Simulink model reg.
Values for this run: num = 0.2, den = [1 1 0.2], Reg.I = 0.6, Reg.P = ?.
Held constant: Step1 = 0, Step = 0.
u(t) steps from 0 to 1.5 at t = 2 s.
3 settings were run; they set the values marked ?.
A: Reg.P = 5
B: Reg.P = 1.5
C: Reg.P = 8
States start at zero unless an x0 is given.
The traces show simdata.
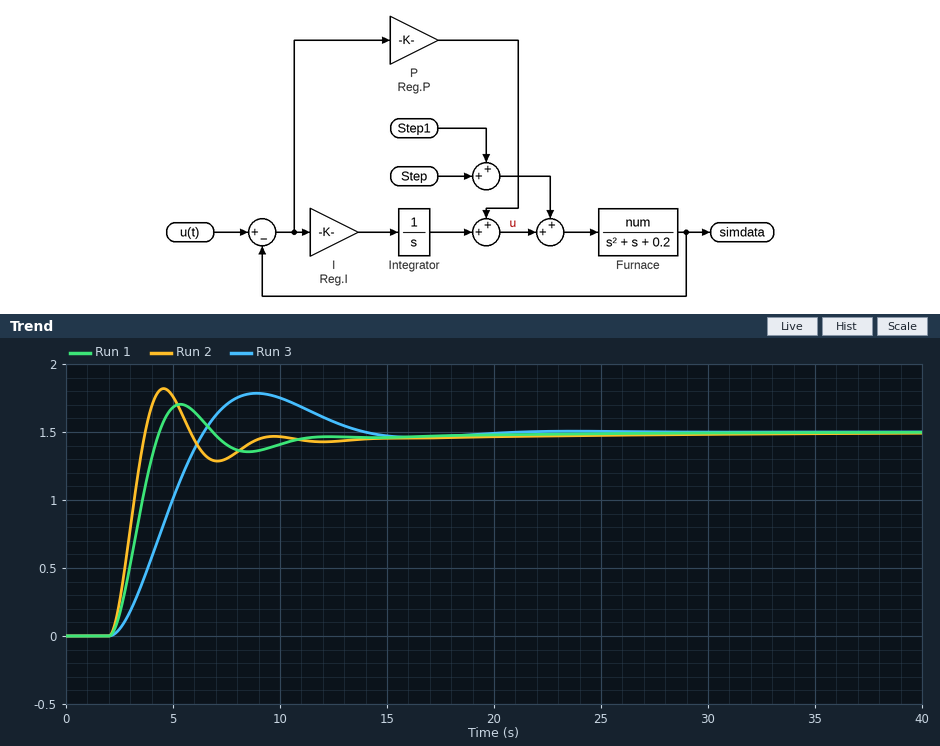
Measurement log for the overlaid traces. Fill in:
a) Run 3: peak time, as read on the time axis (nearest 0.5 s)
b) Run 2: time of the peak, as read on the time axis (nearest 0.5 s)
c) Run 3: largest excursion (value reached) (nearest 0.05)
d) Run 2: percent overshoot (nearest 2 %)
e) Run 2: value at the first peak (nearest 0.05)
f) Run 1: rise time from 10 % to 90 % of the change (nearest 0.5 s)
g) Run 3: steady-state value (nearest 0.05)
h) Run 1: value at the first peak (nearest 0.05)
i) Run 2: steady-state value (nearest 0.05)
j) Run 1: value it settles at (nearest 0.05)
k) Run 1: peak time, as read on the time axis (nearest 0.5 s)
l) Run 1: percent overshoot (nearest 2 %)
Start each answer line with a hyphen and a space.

- 9.0 s
- 4.5 s
- 1.80
- 22 %
- 1.80
- 1.5 s
- 1.50
- 1.70
- 1.50
- 1.50
- 5.5 s
- 14 %
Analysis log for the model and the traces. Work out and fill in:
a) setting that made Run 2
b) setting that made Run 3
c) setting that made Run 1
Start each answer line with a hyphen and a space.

- C
- B
- A
